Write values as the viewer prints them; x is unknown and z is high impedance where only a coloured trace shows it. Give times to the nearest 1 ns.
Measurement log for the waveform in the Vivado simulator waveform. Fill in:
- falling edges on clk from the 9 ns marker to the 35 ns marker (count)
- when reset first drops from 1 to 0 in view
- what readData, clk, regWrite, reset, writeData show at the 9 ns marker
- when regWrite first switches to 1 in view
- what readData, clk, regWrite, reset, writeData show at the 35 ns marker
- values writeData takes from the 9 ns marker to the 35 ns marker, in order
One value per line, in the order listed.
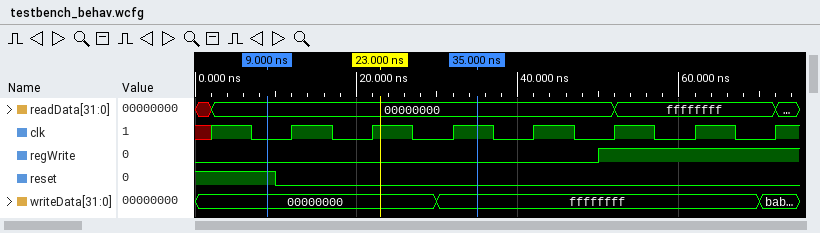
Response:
2
10 ns
readData=00000000, clk=0, regWrite=0, reset=1, writeData=00000000
50 ns
readData=00000000, clk=1, regWrite=0, reset=0, writeData=ffffffff
00000000, ffffffff
